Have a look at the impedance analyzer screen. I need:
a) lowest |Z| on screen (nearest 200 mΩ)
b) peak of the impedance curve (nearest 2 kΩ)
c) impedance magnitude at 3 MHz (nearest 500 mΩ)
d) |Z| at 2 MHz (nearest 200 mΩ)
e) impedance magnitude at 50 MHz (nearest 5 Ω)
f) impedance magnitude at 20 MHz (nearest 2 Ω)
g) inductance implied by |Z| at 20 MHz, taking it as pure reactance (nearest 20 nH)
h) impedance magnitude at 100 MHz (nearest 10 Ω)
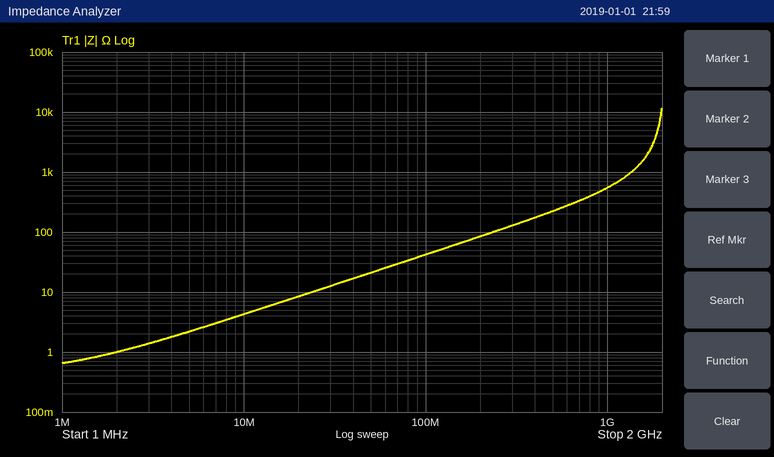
600 mΩ
12 kΩ
1.5 Ω
1.0 Ω
20 Ω
8 Ω
60 nH
40 Ω
